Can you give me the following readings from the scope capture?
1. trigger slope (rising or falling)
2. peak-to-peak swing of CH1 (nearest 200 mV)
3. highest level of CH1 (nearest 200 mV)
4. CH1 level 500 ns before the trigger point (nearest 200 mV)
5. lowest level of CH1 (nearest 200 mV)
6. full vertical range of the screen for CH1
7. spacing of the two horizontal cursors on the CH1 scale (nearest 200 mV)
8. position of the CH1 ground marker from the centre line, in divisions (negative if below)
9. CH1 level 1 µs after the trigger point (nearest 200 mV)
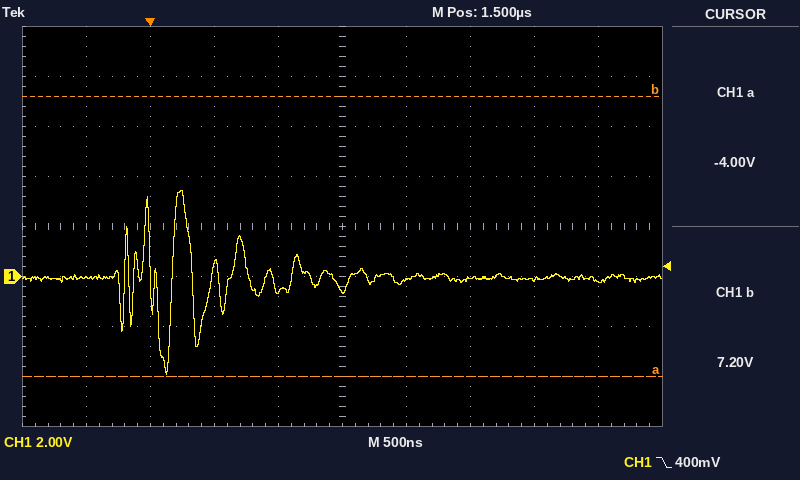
falling
7.4 V
3.4 V
0.0 V
-4.0 V
16 V
11.2 V
-1.0 div
-600 mV
